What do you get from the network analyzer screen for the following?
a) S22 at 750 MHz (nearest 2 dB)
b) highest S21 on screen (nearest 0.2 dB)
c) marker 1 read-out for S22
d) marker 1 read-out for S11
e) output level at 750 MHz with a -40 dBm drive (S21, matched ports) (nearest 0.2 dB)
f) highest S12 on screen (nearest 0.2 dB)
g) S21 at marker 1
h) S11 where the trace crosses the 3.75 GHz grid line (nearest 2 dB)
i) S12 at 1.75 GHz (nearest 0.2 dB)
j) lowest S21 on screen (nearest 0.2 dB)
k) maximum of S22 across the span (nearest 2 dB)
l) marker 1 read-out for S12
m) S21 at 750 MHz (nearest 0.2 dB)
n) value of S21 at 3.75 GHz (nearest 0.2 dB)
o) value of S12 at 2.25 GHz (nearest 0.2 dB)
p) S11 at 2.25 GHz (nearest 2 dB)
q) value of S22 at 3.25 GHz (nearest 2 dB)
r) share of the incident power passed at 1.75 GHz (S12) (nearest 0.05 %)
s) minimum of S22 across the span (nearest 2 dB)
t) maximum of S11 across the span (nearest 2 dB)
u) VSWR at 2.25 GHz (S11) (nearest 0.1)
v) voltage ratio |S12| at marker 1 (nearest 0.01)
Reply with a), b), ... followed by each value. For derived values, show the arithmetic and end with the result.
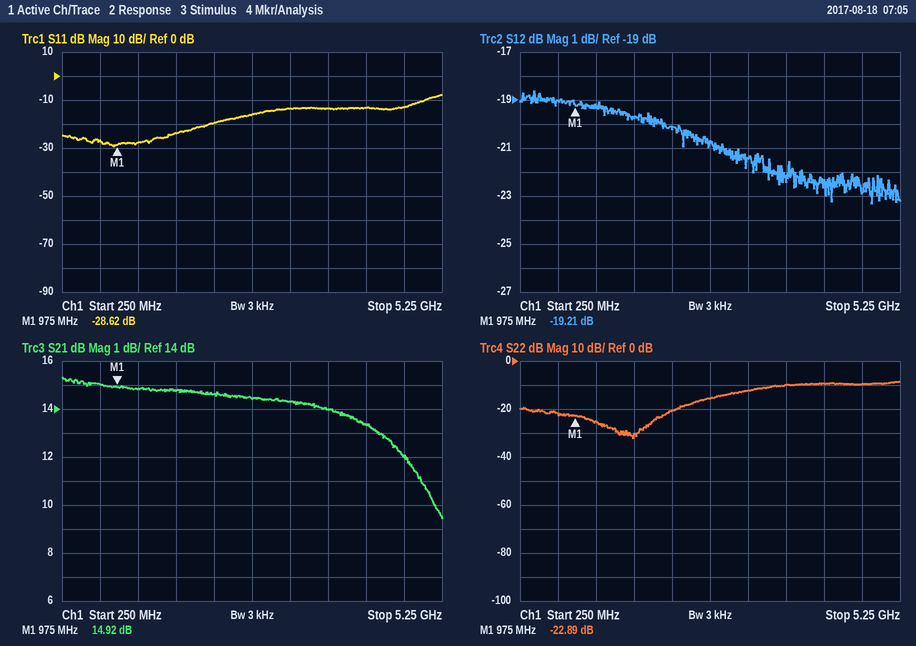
a) -22 dB
b) 15.4 dB
c) -22.89 dB
d) -28.62 dB
e) -40 dBm + (15.0 dB) = -25.0 dBm
f) -18.6 dB
g) 14.92 dB
h) -14 dB
i) -19.8 dB
j) 9.4 dB
k) -8 dB
l) -19.21 dB
m) 15.0 dB
n) 14.0 dB
o) -20.2 dB
p) -20 dB
q) -12 dB
r) 10^(-19.8/10) ≈ 1.05 %
s) -32 dB
t) -8 dB
u) |Γ| = 10^(-20/20) = 0.1000; VSWR = (1 + 0.1000)/(1 − 0.1000) ≈ 1.2
v) 10^(-19.21/20) ≈ 0.11
